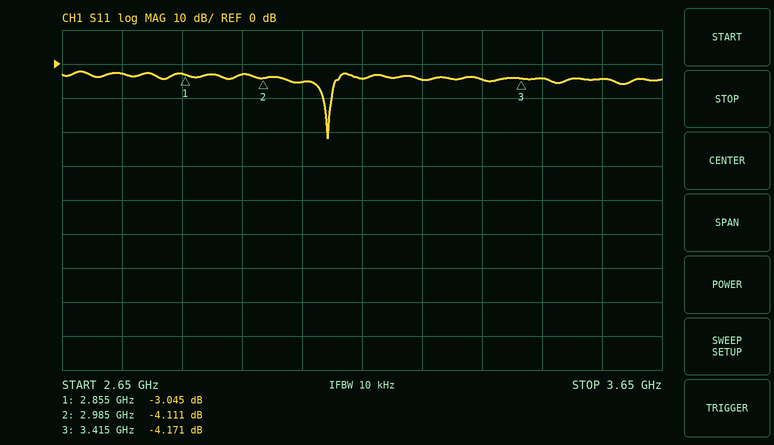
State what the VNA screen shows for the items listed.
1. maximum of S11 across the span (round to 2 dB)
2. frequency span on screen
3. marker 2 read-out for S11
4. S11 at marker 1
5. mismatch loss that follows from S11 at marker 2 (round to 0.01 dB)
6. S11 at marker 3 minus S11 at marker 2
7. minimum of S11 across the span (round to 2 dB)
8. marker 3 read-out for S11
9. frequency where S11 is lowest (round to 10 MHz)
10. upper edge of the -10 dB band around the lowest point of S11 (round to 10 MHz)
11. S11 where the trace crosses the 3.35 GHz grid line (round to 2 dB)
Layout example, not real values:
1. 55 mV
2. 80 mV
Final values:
1. -2 dB
2. 1 GHz
3. -4.111 dB
4. -3.045 dB
5. 2.13 dB
6. -0.060 dB
7. -22 dB
8. -4.171 dB
9. 3.09 GHz
10. 3.10 GHz
11. -4 dB
